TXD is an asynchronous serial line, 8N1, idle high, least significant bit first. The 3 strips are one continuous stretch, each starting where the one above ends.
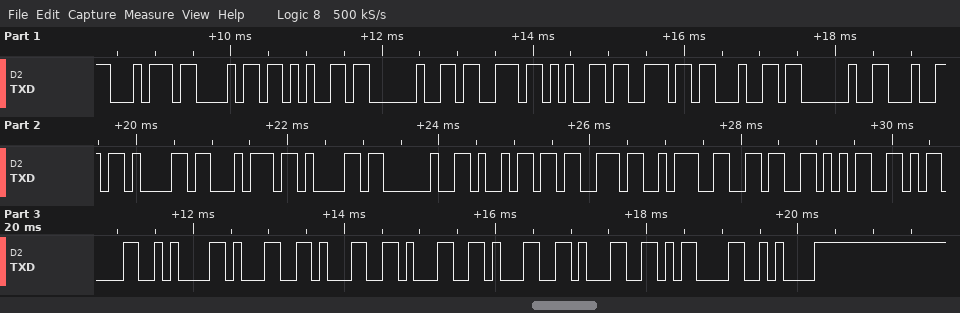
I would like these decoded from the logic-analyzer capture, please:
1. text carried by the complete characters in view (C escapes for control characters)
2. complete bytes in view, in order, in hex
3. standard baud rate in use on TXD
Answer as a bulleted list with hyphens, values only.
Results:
- "the send data is:65\r\n11111\r\n"
- 74 68 65 20 73 65 6E 64 20 64 61 74 61 20 69 73 3A 36 35 0D 0A 31 31 31 31 31 0D 0A
- 9600 baud
